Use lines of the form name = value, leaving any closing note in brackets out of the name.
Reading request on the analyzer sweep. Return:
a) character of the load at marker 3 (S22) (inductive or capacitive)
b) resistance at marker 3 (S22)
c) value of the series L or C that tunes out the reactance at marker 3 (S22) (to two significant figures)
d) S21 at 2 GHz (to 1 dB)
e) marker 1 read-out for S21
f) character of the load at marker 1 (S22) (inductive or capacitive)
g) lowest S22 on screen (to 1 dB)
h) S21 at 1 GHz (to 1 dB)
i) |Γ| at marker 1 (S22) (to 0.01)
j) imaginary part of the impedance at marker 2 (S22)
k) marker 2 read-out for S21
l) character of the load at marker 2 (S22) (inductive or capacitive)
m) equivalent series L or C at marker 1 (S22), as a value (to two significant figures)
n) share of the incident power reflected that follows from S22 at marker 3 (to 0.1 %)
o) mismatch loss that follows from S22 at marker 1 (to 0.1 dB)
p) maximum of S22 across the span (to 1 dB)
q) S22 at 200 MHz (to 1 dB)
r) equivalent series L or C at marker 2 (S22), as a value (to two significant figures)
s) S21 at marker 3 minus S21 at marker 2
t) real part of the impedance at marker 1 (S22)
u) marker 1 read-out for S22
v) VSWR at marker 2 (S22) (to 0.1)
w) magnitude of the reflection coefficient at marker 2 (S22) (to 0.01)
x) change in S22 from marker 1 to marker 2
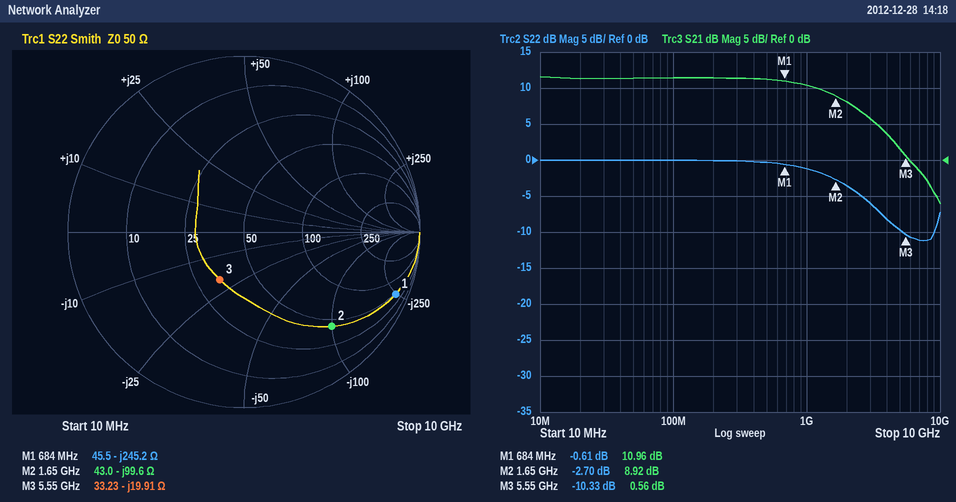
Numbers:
character of the load at marker 3 (S22) = capacitive
resistance at marker 3 = 33.23 Ω
value of the series L or C that tunes out the reactance at marker 3 (S22) = 570 pH
S21 at 2 GHz = 8 dB
marker 1 read-out for S21 = 10.96 dB
character of the load at marker 1 (S22) = capacitive
lowest S22 on screen = -11 dB
S21 at 1 GHz = 10 dB
|Γ| at marker 1 (S22) = 0.93
imaginary part of the impedance at marker 2 = -99.6 Ω
marker 2 read-out for S21 = 8.92 dB
character of the load at marker 2 (S22) = capacitive
equivalent series L or C at marker 1 (S22), as a value = 950 fF
share of the incident power reflected that follows from S22 at marker 3 = 9.3 %
mismatch loss that follows from S22 at marker 1 = 8.8 dB
maximum of S22 across the span = 0 dB
S22 at 200 MHz = 0 dB
equivalent series L or C at marker 2 (S22), as a value = 970 fF
S21 at marker 3 minus S21 at marker 2 = -8.36 dB
real part of the impedance at marker 1 = 45.5 Ω
marker 1 read-out for S22 = -0.61 dB
VSWR at marker 2 (S22) = 6.5
magnitude of the reflection coefficient at marker 2 (S22) = 0.73
change in S22 from marker 1 to marker 2 = -2.09 dB
